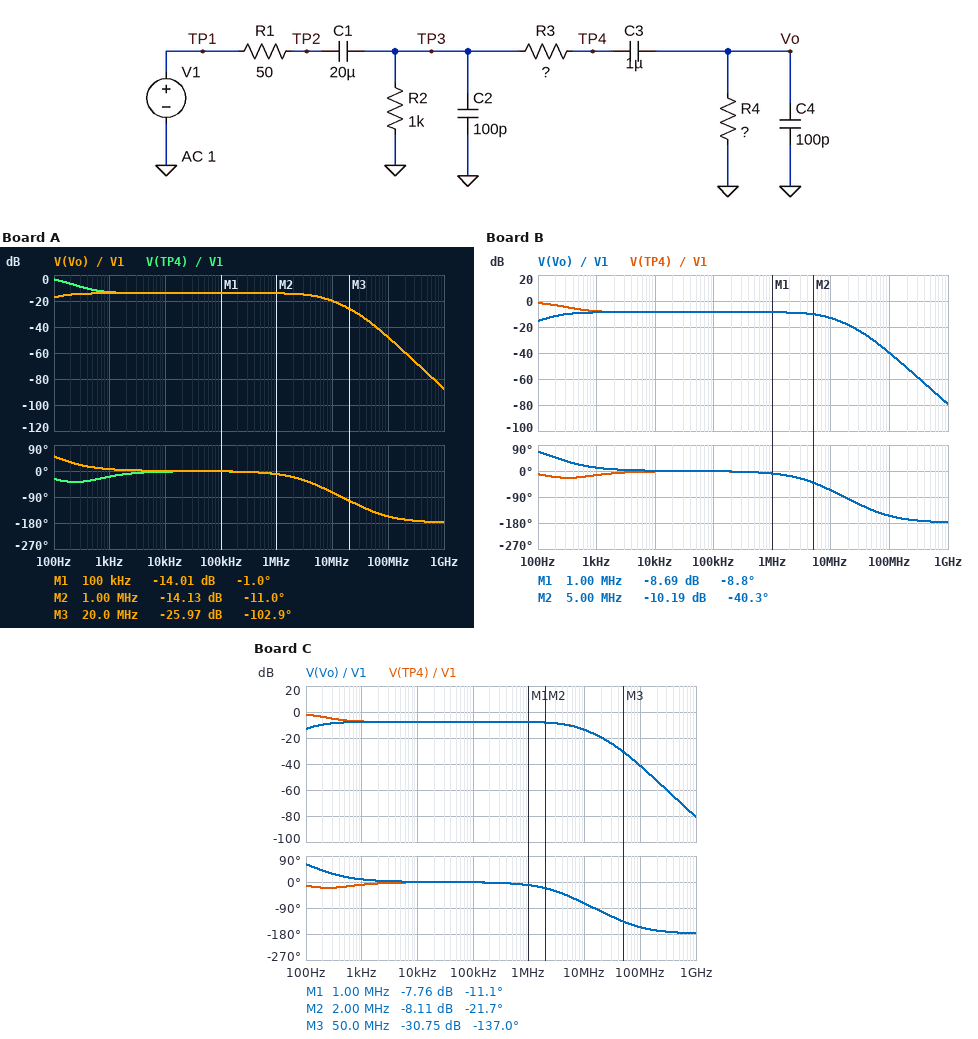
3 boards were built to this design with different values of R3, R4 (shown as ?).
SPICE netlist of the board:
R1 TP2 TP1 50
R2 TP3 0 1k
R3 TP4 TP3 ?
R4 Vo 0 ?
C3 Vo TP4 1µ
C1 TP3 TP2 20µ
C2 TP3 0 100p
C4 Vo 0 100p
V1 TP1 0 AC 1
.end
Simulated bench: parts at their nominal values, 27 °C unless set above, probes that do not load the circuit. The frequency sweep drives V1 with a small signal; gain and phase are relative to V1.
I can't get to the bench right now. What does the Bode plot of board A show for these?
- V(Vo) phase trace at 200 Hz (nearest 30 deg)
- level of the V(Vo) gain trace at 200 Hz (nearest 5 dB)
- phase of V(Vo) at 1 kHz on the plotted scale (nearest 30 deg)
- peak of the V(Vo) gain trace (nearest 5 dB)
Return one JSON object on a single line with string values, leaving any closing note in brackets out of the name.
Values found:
{"V(Vo) phase trace at 200 Hz": "30 deg", "level of the V(Vo) gain trace at 200 Hz": "-15 dB", "phase of V(Vo) at 1 kHz on the plotted scale": "0 deg", "peak of the V(Vo) gain trace": "-15 dB"}
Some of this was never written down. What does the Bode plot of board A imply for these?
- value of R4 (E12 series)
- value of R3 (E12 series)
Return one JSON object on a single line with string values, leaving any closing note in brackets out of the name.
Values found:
{"value of R4": "330 Ω", "value of R3": "1.2 kΩ"}
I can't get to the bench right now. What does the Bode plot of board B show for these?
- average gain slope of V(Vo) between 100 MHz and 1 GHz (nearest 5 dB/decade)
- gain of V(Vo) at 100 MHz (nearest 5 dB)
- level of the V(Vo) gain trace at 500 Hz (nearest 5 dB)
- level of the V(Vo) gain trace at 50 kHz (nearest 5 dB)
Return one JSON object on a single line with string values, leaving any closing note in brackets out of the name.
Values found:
{"average gain slope of V(Vo) between 100 MHz and 1 GHz": "-40 dB/decade", "gain of V(Vo) at 100 MHz": "-40 dB", "level of the V(Vo) gain trace at 500 Hz": "-10 dB", "level of the V(Vo) gain trace at 50 kHz": "-10 dB"}
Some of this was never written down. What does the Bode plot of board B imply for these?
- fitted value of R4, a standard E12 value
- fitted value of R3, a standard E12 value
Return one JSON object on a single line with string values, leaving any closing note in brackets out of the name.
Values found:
{"fitted value of R4, a standard E12 value": "330 Ω", "fitted value of R3, a standard E12 value": "470 Ω"}
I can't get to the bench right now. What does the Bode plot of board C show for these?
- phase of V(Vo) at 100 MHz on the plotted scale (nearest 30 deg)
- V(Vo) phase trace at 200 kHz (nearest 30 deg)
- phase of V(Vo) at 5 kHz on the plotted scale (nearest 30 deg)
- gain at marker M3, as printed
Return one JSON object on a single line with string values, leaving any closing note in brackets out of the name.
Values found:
{"phase of V(Vo) at 100 MHz on the plotted scale": "-150 deg", "V(Vo) phase trace at 200 kHz": "0 deg", "phase of V(Vo) at 5 kHz on the plotted scale": "0 deg", "gain at marker M3, as printed": "-30.75 dB"}
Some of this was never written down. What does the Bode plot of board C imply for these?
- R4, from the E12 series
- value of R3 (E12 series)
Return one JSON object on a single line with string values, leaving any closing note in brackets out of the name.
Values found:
{"R4, from the E12 series": "470 Ω", "value of R3": "560 Ω"}
